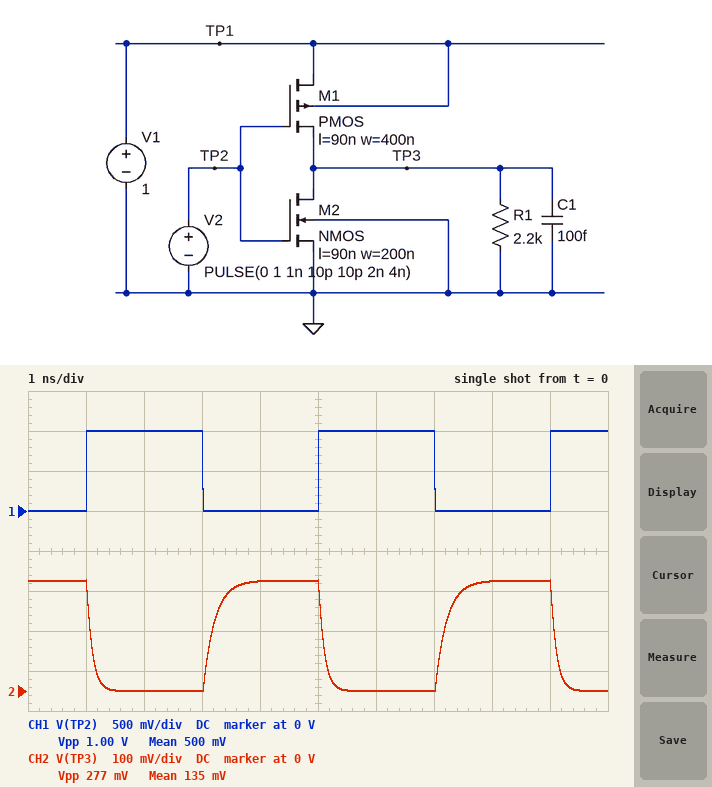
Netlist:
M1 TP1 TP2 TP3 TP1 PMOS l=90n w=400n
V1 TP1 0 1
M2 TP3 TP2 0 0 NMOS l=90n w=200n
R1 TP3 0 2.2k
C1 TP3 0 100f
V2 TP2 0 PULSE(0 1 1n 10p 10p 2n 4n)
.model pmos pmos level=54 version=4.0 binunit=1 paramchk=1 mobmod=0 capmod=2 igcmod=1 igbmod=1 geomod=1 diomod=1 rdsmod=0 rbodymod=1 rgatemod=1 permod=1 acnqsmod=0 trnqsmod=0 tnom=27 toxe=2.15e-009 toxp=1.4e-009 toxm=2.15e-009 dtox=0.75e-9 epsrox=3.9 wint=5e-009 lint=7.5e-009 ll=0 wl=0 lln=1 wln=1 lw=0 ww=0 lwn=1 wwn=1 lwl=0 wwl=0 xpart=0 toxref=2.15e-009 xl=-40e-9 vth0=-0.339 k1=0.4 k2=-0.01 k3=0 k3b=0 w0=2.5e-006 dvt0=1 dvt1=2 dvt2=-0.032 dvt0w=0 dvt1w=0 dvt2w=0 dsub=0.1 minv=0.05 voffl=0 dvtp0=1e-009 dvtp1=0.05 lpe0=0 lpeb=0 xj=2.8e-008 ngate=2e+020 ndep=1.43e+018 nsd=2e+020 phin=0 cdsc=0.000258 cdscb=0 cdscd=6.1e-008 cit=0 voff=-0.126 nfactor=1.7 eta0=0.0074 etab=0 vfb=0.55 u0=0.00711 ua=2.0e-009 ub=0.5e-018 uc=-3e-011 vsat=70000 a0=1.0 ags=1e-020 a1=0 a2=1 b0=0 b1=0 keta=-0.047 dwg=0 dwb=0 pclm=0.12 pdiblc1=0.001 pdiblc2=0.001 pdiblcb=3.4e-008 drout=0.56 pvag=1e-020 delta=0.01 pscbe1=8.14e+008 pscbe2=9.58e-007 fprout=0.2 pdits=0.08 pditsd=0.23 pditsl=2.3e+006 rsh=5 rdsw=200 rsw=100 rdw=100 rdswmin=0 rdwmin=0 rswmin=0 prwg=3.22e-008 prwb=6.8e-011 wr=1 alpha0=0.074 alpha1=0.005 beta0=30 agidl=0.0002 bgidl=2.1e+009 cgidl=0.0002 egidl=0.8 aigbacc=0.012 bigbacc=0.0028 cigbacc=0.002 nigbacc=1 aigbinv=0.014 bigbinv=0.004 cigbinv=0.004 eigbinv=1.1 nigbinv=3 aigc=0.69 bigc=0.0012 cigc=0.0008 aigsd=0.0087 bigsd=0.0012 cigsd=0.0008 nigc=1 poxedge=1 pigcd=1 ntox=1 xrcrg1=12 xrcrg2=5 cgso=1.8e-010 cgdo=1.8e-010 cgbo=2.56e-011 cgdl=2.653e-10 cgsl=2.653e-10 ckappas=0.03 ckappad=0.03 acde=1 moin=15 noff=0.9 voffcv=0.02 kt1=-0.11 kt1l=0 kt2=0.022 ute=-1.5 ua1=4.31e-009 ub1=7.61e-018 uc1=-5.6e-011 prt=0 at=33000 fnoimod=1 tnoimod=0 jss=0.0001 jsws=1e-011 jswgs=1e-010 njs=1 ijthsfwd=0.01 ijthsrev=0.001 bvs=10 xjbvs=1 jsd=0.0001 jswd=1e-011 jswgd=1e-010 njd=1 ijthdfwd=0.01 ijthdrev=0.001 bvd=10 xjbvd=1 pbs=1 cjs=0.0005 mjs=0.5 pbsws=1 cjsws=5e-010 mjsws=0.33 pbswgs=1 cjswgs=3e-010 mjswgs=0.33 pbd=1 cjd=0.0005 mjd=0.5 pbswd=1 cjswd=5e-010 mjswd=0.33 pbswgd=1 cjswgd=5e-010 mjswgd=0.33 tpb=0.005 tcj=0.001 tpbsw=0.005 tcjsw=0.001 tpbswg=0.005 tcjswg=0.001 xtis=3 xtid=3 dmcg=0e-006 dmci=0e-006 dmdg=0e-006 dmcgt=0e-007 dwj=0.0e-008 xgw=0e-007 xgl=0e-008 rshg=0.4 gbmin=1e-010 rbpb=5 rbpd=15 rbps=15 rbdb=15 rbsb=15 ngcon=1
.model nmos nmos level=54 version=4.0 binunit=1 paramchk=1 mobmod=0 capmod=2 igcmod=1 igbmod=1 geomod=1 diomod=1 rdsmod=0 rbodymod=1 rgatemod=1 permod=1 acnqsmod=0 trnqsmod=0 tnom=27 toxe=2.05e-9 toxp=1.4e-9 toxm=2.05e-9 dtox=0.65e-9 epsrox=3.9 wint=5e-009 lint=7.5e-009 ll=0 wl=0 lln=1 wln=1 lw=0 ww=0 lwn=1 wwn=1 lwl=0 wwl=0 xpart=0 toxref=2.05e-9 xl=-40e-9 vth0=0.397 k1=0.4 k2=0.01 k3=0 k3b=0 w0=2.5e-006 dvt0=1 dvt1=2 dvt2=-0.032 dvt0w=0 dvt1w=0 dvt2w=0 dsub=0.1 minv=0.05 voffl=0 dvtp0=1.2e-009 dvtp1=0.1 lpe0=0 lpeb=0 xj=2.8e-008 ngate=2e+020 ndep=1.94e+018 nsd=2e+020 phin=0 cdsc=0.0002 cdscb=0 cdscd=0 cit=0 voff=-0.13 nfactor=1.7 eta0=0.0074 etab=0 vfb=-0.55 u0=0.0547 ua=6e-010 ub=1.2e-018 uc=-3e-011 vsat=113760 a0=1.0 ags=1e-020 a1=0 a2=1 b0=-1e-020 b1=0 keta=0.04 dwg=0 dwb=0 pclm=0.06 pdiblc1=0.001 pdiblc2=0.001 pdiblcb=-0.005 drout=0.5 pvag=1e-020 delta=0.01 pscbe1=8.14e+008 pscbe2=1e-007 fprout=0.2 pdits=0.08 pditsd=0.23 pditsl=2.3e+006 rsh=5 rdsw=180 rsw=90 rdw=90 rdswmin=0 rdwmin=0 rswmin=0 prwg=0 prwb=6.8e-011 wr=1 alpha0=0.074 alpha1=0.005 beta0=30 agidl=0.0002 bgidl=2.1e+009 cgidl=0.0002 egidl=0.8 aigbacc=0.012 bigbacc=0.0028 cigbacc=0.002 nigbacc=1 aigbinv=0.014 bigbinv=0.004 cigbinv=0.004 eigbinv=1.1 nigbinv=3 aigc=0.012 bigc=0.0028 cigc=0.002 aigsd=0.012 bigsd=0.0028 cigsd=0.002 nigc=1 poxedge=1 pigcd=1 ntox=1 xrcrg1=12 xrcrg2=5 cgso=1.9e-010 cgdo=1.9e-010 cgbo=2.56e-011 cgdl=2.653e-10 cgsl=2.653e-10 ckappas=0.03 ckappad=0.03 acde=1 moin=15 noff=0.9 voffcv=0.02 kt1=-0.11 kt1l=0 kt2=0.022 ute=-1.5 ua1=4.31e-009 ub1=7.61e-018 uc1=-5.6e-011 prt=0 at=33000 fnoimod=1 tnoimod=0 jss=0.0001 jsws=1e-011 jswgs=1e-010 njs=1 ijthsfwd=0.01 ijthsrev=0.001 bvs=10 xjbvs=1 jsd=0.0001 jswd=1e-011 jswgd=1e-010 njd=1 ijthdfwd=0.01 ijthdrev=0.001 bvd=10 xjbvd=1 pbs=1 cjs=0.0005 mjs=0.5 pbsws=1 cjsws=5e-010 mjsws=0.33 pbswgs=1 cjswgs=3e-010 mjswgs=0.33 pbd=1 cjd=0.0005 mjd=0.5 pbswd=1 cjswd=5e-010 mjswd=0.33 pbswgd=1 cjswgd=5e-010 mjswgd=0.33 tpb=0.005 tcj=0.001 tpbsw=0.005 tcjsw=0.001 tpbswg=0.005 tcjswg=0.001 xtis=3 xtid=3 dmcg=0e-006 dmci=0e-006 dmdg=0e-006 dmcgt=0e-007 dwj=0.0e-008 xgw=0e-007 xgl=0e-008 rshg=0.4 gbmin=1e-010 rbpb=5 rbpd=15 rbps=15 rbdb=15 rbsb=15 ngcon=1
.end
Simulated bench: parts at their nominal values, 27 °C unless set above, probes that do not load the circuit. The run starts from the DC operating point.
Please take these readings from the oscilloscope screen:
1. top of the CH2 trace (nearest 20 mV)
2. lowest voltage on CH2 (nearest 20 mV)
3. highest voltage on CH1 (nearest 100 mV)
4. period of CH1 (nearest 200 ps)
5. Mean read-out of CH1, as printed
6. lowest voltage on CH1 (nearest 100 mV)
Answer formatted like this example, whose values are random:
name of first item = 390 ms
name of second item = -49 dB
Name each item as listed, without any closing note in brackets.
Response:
top of the CH2 trace = 280 mV
lowest voltage on CH2 = 0 V
highest voltage on CH1 = 1.0 V
period of CH1 = 4.0 ns
Mean read-out of CH1, as printed = 500 mV
lowest voltage on CH1 = 0 V
